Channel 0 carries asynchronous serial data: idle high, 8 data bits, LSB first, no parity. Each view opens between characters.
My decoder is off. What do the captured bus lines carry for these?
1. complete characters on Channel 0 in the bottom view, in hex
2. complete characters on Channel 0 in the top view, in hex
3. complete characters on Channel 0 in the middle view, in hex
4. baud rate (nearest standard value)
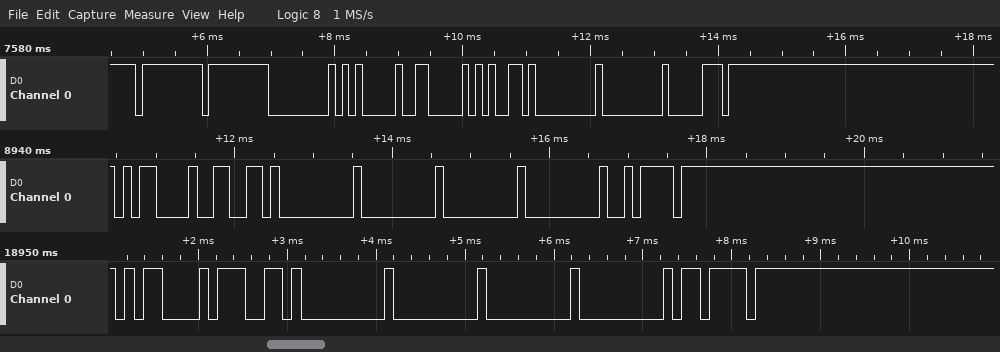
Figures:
0D, 67, 00, 00, 00, 00, 7B
FF, FF, 00, 05, 06, 65, 00, 00, 70
0D, 66, 00, 00, 00, 00, 7A
9600 baud
